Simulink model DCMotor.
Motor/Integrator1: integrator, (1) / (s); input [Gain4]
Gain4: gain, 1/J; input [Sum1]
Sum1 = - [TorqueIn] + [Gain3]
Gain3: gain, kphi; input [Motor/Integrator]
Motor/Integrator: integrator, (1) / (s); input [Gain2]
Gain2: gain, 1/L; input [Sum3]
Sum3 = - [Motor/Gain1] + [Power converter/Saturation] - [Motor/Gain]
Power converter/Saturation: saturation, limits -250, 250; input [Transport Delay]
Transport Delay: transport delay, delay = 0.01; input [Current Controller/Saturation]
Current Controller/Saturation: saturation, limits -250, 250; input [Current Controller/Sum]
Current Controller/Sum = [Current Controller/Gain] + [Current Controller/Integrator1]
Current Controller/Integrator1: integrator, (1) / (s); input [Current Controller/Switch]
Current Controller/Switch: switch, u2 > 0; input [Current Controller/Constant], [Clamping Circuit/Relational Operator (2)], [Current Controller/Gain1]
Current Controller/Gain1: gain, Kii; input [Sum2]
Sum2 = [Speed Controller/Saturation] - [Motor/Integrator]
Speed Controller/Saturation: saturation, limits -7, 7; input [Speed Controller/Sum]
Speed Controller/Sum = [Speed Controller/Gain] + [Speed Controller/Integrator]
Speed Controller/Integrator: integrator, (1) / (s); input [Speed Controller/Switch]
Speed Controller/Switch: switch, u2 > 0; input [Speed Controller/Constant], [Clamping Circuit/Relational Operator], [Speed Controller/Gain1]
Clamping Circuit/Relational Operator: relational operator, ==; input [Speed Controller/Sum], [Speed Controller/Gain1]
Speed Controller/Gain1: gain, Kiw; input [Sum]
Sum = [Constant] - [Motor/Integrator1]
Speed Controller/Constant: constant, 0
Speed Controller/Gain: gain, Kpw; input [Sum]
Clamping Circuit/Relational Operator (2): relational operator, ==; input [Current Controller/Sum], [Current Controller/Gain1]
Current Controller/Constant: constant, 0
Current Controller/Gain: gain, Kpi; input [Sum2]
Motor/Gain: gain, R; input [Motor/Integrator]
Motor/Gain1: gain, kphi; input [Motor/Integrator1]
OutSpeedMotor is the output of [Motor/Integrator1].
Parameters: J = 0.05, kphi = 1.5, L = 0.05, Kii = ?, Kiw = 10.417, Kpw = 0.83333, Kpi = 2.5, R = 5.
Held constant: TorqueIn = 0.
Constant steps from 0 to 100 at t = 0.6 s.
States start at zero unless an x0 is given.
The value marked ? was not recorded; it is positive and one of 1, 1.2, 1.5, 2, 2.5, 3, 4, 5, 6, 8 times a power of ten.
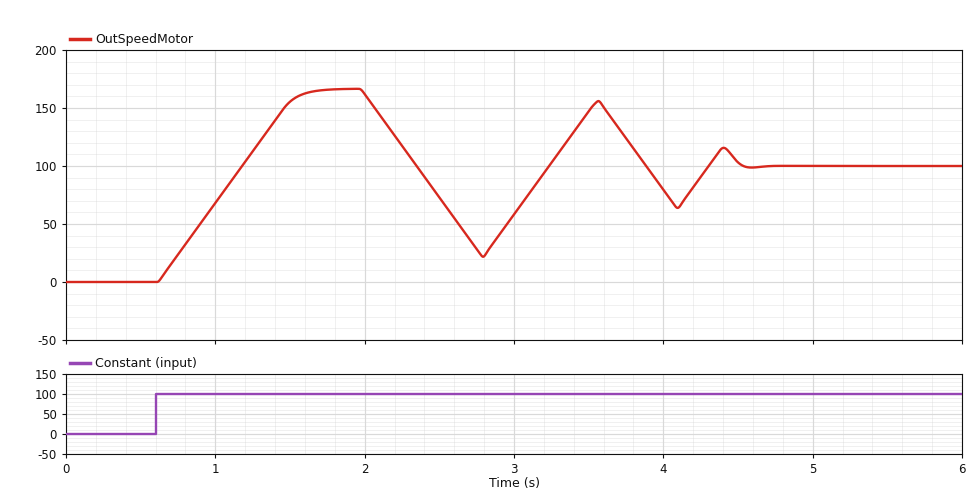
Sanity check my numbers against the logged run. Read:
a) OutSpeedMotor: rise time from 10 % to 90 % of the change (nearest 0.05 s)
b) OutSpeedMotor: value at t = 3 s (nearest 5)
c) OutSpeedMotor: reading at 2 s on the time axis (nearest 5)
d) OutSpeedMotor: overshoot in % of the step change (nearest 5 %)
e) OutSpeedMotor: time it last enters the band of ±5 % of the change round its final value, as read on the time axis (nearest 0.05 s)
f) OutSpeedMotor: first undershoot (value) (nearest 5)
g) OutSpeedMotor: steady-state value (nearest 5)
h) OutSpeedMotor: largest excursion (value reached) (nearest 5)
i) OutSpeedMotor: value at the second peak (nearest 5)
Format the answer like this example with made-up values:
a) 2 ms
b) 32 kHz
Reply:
a) 0.45 s
b) 60
c) 160
d) 65 %
e) 4.50 s
f) 20
g) 100
h) 165
i) 155
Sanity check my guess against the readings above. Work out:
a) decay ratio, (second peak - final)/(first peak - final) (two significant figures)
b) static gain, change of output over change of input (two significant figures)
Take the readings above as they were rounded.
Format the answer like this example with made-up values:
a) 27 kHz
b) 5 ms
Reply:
a) 0.85
b) 1.0
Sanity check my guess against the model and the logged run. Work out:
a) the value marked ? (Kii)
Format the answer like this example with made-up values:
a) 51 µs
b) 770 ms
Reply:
a) 250
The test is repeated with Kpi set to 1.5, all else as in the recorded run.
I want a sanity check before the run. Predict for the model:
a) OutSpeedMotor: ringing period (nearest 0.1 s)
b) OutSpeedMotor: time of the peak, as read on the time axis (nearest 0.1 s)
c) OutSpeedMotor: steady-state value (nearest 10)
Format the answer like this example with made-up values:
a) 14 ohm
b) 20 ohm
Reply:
a) 1.6 s
b) 2.0 s
c) 100
